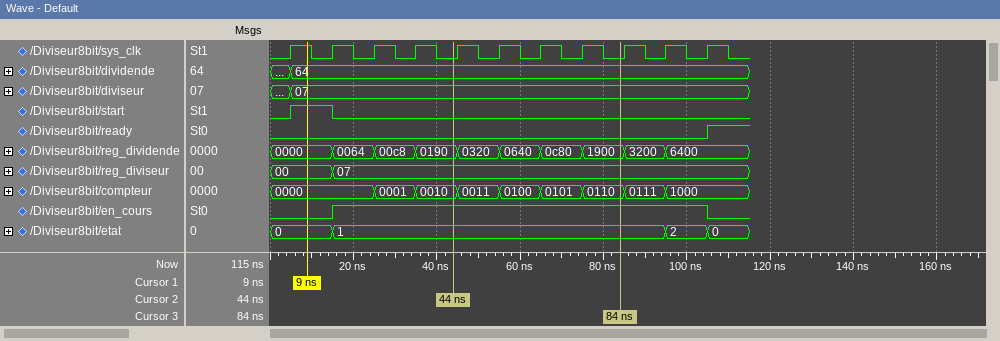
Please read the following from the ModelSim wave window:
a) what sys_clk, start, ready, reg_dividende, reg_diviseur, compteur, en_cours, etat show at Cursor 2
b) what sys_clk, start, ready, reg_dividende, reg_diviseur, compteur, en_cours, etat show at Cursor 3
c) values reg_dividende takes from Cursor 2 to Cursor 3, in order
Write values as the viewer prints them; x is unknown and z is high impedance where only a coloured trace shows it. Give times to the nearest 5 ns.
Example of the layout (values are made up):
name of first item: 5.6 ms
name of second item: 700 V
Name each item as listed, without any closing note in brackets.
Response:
what sys_clk, start, ready, reg_dividende, reg_diviseur, compteur, en_cours, etat show at Cursor 2: sys_clk=0, start=0, ready=0, reg_dividende=0190, reg_diviseur=07, compteur=0010, en_cours=1, etat=1
what sys_clk, start, ready, reg_dividende, reg_diviseur, compteur, en_cours, etat show at Cursor 3: sys_clk=0, start=0, ready=0, reg_dividende=1900, reg_diviseur=07, compteur=0110, en_cours=1, etat=1
values reg_dividende takes from Cursor 2 to Cursor 3, in order: 0190, 0320, 0640, 0c80, 1900
